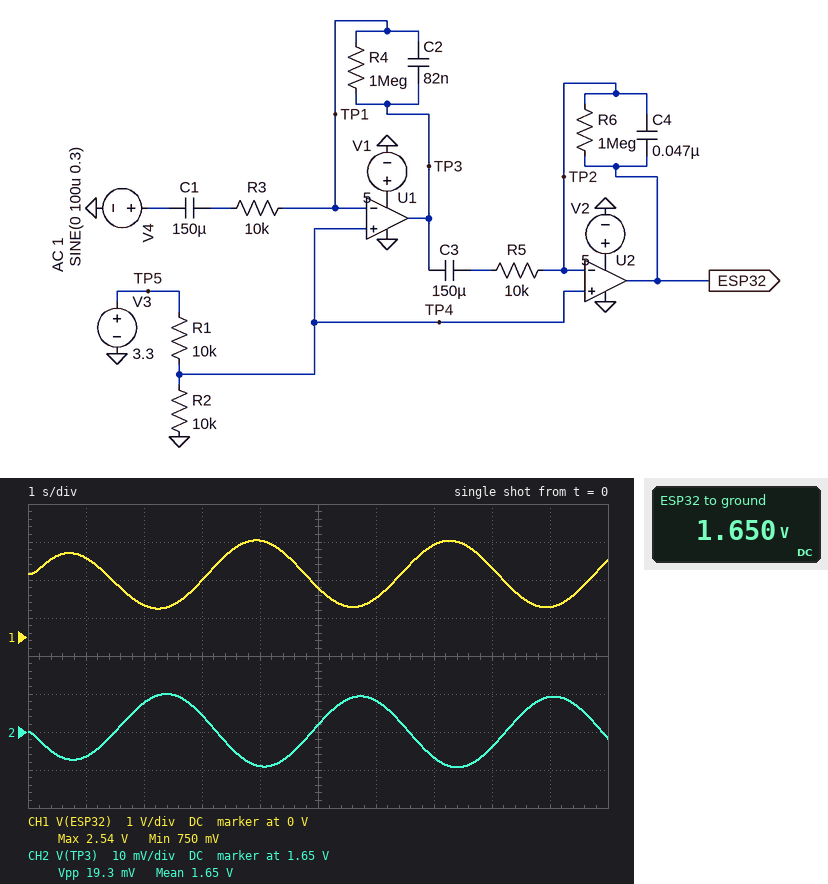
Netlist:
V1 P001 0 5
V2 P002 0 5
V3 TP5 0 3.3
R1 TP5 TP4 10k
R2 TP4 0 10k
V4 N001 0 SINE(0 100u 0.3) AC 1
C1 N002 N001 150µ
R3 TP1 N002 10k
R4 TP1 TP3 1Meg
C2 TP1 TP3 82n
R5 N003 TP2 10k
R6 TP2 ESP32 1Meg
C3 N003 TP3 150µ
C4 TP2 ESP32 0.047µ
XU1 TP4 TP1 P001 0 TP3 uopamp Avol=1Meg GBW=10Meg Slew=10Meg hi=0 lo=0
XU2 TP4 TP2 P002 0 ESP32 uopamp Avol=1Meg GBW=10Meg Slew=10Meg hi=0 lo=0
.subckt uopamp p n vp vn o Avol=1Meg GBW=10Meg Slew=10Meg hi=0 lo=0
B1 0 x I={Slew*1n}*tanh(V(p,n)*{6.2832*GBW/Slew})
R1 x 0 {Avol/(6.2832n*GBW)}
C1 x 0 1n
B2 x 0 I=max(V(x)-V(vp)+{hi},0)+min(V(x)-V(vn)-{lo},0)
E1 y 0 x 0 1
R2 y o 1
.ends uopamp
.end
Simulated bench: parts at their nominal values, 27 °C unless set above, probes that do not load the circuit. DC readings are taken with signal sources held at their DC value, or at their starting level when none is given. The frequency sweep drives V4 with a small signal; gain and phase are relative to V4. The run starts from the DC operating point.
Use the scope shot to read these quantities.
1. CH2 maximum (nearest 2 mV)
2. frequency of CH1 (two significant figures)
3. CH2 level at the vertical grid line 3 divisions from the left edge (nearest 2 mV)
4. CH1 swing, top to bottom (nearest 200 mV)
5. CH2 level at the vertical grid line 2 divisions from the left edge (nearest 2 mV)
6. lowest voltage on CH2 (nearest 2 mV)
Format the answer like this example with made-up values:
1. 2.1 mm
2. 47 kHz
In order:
1. 1.660 V
2. 300 mHz
3. 1.654 V
4. 1.8 V
5. 1.658 V
6. 1.640 V
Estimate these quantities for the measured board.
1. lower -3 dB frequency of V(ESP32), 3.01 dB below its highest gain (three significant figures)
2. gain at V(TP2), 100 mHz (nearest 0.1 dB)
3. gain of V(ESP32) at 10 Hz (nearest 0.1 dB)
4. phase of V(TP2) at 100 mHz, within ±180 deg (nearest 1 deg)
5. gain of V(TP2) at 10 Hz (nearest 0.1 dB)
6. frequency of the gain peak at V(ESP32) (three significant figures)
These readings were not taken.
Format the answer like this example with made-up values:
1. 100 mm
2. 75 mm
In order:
1. 145 mHz
2. -46.6 dB
3. 55.7 dB
4. -91 deg
5. -61.3 dB
6. 504 mHz
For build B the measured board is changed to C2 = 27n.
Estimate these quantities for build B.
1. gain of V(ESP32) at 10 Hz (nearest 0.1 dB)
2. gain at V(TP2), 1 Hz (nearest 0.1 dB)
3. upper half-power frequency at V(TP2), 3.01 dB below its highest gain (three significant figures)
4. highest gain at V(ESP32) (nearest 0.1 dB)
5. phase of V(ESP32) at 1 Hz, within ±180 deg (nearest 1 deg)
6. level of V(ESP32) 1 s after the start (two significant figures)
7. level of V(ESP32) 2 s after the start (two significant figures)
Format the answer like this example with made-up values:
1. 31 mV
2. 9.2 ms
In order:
1. 64.2 dB
2. -40.5 dB
3. 3.17 Hz
4. 79.6 dB
5. -14 deg
6. 2.0 V
7. 790 mV
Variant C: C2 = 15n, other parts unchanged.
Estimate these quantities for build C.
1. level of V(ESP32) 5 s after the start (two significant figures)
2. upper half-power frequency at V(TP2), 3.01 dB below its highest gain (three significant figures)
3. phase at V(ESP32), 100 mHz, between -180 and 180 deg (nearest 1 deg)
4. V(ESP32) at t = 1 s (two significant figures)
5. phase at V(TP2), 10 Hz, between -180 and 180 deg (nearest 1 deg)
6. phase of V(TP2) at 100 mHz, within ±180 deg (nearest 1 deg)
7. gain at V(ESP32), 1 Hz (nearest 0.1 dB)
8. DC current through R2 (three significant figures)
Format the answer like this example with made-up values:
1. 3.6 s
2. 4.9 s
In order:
1. 1.2 V
2. 3.72 Hz
3. 91 deg
4. 2.0 V
5. 112 deg
6. -88 deg
7. 79.5 dB
8. 165 µA
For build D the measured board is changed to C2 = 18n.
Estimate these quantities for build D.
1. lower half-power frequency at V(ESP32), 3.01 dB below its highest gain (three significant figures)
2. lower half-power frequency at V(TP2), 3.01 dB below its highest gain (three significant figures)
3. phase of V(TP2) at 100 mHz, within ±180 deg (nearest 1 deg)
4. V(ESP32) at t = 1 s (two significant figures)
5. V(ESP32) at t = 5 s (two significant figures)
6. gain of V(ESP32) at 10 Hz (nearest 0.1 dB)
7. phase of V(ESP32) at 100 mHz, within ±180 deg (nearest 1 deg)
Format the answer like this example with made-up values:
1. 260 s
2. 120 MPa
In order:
1. 153 mHz
2. 154 mHz
3. -88 deg
4. 2.0 V
5. 1.2 V
6. 66.5 dB
7. 91 deg
